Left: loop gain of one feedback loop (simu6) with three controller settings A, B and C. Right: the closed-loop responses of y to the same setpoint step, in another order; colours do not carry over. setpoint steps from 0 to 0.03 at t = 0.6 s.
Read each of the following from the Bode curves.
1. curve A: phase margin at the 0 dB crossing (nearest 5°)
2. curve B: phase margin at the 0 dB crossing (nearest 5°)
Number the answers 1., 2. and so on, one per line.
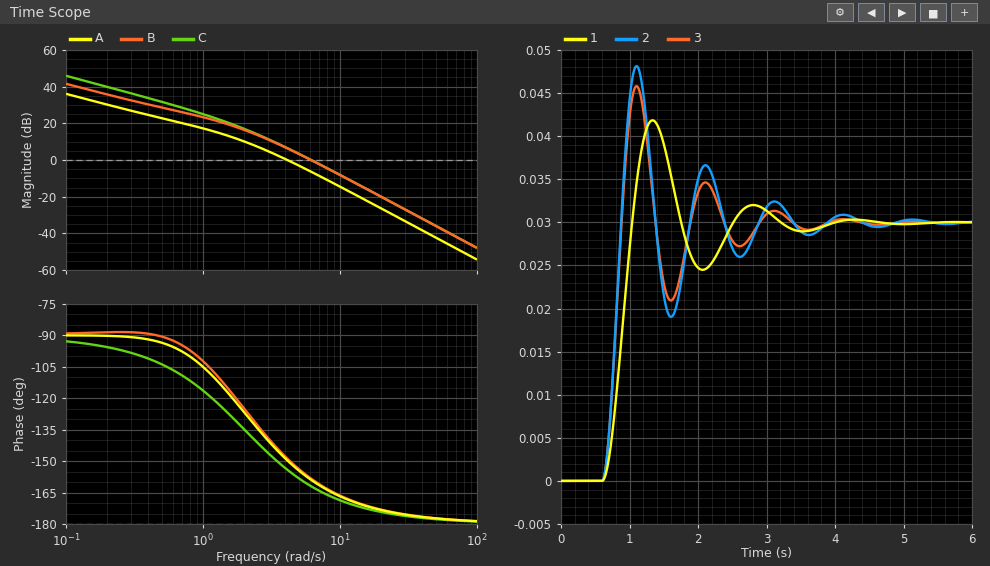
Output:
1. 30°
2. 20°
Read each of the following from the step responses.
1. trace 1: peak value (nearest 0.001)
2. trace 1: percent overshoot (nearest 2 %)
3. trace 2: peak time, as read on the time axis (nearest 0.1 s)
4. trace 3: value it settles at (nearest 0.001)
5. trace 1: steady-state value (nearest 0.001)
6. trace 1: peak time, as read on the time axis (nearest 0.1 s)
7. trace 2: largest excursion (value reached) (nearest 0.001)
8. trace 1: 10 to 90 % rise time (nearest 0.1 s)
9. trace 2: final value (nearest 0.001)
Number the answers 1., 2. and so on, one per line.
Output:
1. 0.042
2. 40 %
3. 1.1 s
4. 0.030
5. 0.030
6. 1.3 s
7. 0.048
8. 0.3 s
9. 0.030
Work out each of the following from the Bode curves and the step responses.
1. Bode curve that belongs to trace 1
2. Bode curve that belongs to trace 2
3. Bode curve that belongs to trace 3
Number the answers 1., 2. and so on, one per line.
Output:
1. A
2. C
3. B
